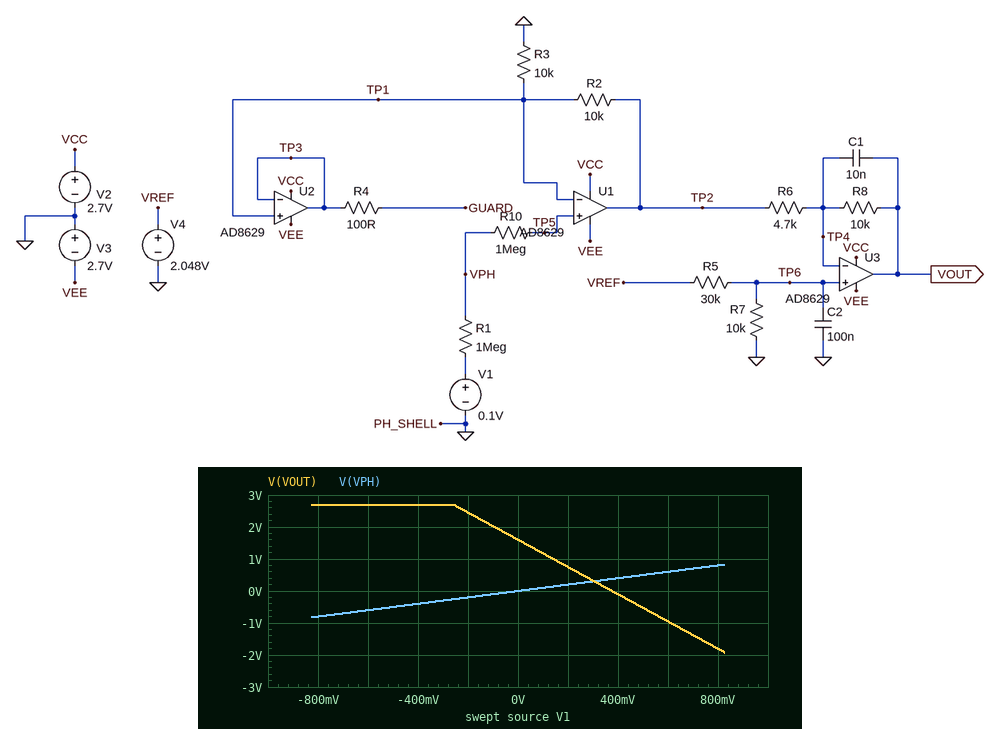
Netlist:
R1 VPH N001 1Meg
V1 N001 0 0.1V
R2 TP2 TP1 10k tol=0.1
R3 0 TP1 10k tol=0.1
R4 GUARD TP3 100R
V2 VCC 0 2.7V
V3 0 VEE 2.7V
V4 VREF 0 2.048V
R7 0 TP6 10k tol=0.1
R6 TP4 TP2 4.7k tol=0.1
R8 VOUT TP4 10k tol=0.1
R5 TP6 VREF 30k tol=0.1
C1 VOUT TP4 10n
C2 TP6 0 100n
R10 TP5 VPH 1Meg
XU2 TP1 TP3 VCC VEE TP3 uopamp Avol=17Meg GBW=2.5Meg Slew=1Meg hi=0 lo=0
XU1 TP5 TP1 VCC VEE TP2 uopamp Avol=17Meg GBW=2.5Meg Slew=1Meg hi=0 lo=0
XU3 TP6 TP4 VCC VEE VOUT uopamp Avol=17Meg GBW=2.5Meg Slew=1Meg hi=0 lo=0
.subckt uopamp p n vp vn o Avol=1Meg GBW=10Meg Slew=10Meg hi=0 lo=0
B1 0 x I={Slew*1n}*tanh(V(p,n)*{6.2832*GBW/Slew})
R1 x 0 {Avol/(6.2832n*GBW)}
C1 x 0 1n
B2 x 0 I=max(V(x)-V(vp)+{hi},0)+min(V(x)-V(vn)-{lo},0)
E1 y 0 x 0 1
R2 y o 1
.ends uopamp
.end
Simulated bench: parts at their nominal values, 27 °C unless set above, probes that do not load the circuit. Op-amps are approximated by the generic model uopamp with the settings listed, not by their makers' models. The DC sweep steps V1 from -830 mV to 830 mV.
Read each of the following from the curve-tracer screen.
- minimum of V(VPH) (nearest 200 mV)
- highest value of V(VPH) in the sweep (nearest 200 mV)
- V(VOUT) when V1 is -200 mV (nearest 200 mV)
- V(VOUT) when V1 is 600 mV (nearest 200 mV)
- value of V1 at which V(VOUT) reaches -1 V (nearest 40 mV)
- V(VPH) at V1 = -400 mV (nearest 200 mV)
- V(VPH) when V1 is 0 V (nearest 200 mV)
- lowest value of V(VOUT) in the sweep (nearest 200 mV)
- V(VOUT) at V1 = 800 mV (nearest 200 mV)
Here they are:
-800 mV
800 mV
2.4 V
-1.0 V
600 mV
-400 mV
0 V
-2.0 V
-1.8 V
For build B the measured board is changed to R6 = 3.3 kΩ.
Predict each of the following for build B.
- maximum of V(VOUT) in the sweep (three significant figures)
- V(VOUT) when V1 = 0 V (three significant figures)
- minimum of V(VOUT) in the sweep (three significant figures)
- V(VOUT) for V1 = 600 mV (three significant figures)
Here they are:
2.70 V
2.06 V
-2.70 V
-1.57 V
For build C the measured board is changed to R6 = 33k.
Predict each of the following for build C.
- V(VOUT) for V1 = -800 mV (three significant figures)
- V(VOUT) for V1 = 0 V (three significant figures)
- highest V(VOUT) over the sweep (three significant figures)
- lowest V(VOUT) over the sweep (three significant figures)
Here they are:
1.15 V
667 mV
1.17 V
164 mV
